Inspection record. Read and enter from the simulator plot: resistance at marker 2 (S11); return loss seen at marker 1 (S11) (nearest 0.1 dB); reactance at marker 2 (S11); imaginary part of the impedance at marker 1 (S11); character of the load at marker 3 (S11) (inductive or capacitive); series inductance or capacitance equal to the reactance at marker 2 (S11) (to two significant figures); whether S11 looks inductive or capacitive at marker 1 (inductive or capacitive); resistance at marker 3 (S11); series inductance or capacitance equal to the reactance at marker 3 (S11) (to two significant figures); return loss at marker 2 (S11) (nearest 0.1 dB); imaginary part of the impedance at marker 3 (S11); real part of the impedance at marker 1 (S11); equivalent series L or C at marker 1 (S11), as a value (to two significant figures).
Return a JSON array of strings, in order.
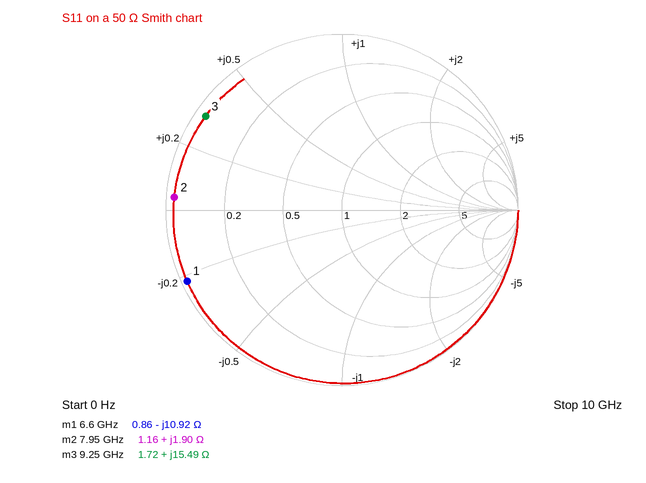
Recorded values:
["1.16 Ω", "0.3 dB", "+1.90 Ω", "-10.92 Ω", "inductive", "38 pH", "capacitive", "1.72 Ω", "270 pH", "0.4 dB", "+15.49 Ω", "0.86 Ω", "2.2 pF"]
